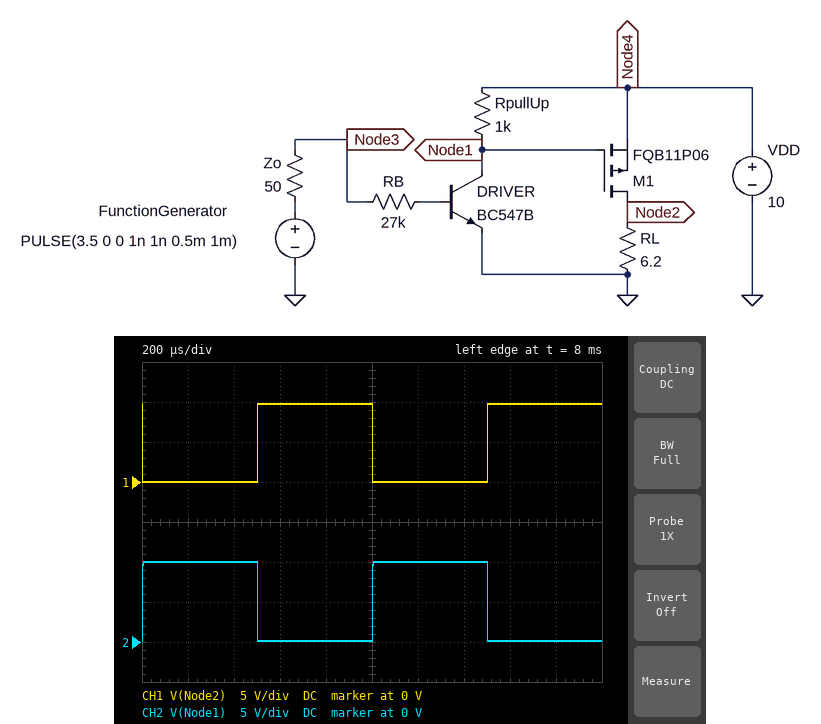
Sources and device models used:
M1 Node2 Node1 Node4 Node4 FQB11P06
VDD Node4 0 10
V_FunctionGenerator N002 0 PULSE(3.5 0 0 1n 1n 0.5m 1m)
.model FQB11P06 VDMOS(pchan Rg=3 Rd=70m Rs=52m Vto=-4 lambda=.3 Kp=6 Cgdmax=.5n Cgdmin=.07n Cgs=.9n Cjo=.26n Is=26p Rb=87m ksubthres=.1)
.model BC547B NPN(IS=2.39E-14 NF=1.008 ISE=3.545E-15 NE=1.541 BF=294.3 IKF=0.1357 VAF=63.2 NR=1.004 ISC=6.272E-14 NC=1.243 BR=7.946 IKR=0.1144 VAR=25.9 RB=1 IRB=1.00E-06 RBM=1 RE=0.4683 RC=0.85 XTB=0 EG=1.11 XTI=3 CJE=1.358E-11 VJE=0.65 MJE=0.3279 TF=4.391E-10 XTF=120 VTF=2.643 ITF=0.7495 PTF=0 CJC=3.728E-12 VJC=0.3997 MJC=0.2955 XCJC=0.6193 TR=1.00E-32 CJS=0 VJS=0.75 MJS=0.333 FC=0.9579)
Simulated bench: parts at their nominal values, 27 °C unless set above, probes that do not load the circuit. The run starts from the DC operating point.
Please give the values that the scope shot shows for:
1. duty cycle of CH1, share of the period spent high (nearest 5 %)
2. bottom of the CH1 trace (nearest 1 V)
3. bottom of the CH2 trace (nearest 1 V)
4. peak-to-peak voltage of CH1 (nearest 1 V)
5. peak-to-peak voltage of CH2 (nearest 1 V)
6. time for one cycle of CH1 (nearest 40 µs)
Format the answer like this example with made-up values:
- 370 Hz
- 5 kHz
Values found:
- 50 %
- 0 V
- 0 V
- 10 V
- 10 V
- 1.00 ms
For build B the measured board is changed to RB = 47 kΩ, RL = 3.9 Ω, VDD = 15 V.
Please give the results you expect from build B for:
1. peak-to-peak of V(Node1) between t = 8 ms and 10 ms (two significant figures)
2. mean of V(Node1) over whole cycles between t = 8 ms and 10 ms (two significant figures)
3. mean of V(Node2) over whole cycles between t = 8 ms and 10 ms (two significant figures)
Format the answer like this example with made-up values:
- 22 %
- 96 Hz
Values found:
- 15 V
- 7.6 V
- 7.3 V
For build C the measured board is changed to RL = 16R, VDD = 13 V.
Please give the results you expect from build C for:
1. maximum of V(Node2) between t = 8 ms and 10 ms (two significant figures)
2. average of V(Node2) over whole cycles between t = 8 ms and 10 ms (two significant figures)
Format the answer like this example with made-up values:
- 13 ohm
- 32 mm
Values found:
- 13 V
- 6.5 V
